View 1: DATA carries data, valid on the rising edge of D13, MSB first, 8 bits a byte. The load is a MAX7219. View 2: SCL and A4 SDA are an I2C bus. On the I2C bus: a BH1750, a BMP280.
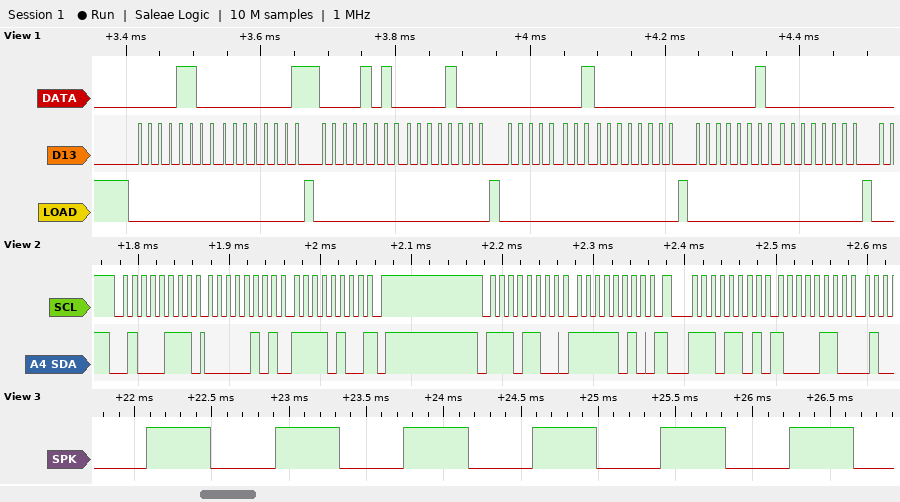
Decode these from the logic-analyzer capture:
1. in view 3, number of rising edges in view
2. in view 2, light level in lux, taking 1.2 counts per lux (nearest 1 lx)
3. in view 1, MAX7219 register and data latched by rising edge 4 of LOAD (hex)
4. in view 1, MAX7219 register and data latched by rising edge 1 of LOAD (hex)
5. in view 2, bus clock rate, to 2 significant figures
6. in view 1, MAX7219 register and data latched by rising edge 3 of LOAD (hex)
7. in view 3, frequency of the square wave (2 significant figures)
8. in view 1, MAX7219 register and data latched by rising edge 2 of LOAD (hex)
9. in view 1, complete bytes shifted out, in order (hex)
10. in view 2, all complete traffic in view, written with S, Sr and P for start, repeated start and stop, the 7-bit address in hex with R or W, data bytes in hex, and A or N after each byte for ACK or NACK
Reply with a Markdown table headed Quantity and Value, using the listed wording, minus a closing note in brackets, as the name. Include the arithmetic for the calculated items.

| Quantity | Value |
|---|---|
| in view 3, number of rising edges in view | 6 |
| in view 2, light level in lux, taking 1.2 counts per lux | 1524 / 1.2 = 1270 lx |
| in view 1, MAX7219 register and data latched by rising edge 4 of LOAD | register 0x2, data 0x00 |
| in view 1, MAX7219 register and data latched by rising edge 1 of LOAD | register 0xC, data 0x01 |
| in view 2, bus clock rate, to 2 significant figures | 100 kHz |
| in view 1, MAX7219 register and data latched by rising edge 3 of LOAD | register 0x1, data 0x00 |
| in view 3, frequency of the square wave | 1.2 kHz |
| in view 1, MAX7219 register and data latched by rising edge 2 of LOAD | register 0xA, data 0x08 |
| in view 1, complete bytes shifted out, in order | 0x0C 0x01 0x0A 0x08 0x01 0x00 0x02 0x00 |
| in view 2, all complete traffic in view, written with S, Sr and P for start, repeated start and stop, the 7-bit address in hex with R or W, data bytes in hex, and A or N after each byte for ACK or NACK | S 23R A 05 A F4 N P S 76W A FA A Sr 76R A 86 A |
